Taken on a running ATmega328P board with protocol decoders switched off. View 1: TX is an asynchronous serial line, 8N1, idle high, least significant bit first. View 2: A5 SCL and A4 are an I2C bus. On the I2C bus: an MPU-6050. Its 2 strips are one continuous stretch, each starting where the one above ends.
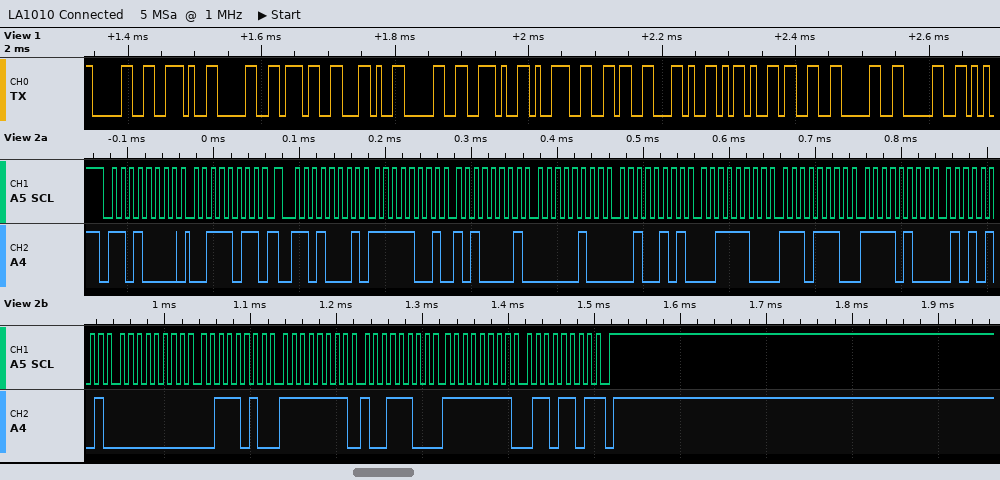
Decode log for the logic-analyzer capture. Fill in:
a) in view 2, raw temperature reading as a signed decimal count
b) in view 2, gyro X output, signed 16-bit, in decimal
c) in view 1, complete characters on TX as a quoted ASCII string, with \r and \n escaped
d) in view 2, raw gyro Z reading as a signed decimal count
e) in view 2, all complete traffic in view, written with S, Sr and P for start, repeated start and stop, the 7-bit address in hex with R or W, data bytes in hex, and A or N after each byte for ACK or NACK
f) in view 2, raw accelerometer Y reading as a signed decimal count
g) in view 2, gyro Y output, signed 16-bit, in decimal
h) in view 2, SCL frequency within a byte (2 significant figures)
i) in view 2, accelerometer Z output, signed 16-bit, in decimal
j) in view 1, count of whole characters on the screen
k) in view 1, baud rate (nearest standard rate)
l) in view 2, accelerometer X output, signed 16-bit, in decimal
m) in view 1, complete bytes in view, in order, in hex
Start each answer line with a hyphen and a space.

- -2987
- 58
- "0.07,0.96,-300"
- -147
- S 68W A 3B A Sr 68R A F9 A A1 A 04 A 25 A 3C A EE A F4 A 55 A 00 A 3A A FF A 9C A FF A 6D N P
- 1061
- -100
- 100 kHz
- 15598
- 14
- 115200 baud
- -1631
- 0x30 0x2E 0x30 0x37 0x2C 0x30 0x2E 0x39 0x36 0x2C 0x2D 0x33 0x30 0x30
